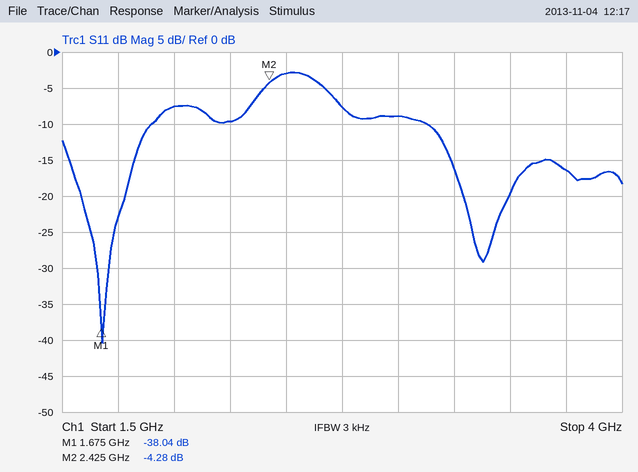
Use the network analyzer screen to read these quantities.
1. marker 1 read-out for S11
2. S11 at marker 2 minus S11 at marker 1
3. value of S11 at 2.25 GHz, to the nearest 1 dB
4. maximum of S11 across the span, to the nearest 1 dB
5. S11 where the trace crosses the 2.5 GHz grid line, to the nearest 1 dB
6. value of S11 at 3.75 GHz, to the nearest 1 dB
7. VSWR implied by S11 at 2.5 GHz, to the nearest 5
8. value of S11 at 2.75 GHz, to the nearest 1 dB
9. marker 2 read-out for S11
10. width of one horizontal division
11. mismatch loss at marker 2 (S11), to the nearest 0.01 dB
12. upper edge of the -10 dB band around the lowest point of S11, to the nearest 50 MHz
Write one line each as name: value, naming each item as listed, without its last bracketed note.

marker 1 read-out for S11: -38.04 dB
S11 at marker 2 minus S11 at marker 1: 33.76 dB
value of S11 at 2.25 GHz, to the nearest 1 dB: -10 dB
maximum of S11 across the span, to the nearest 1 dB: -3 dB
S11 where the trace crosses the 2.5 GHz grid line, to the nearest 1 dB: -3 dB
value of S11 at 3.75 GHz, to the nearest 1 dB: -16 dB
VSWR implied by S11 at 2.5 GHz, to the nearest 5: 5
value of S11 at 2.75 GHz, to the nearest 1 dB: -8 dB
marker 2 read-out for S11: -4.28 dB
width of one horizontal division: 250 MHz
mismatch loss at marker 2 (S11), to the nearest 0.01 dB: 2.03 dB
upper edge of the -10 dB band around the lowest point of S11, to the nearest 50 MHz: 1.90 GHz
